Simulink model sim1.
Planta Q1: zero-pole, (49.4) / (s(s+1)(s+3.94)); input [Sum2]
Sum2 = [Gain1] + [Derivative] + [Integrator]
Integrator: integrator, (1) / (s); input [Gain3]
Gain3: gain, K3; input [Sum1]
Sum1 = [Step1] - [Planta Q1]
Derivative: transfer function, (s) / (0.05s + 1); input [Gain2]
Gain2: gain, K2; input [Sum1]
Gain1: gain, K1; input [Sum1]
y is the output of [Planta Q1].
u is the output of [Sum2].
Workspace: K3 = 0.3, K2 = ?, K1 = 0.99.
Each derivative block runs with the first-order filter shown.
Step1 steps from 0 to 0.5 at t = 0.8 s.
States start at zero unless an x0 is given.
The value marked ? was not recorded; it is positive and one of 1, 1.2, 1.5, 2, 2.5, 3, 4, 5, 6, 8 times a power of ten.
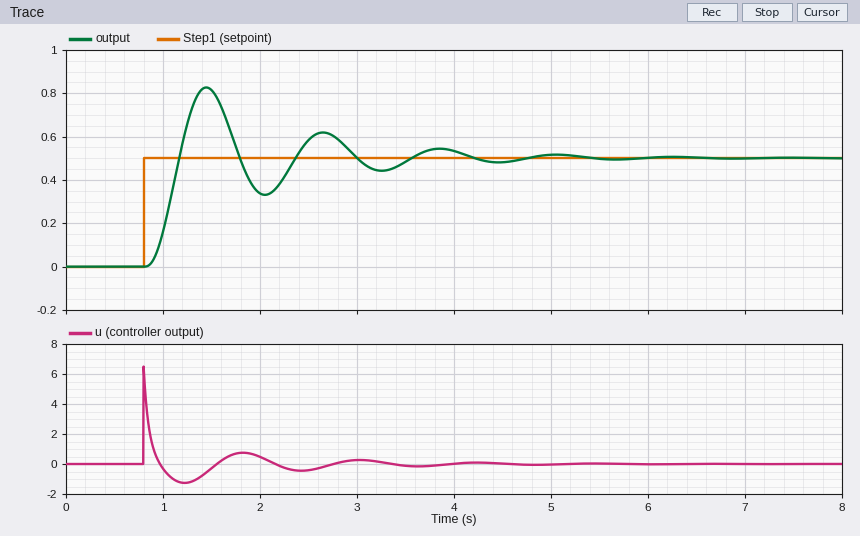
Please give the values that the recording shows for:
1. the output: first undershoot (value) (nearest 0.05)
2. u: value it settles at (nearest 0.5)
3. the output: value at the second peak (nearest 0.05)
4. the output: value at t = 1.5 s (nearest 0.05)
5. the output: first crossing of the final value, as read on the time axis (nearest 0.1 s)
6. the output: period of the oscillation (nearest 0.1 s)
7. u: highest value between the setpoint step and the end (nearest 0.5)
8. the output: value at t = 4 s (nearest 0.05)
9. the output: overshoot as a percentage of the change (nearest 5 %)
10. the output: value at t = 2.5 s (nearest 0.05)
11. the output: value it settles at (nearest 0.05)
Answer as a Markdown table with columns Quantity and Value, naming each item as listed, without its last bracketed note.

| Quantity | Value |
|---|---|
| the output: first undershoot (value) | 0.35 |
| u: value it settles at | 0.0 |
| the output: value at the second peak | 0.60 |
| the output: value at t = 1.5 s | 0.80 |
| the output: first crossing of the final value, as read on the time axis | 1.2 s |
| the output: period of the oscillation | 1.2 s |
| u: highest value between the setpoint step and the end | 6.5 |
| the output: value at t = 4 s | 0.55 |
| the output: overshoot as a percentage of the change | 65 % |
| the output: value at t = 2.5 s | 0.60 |
| the output: value it settles at | 0.50 |
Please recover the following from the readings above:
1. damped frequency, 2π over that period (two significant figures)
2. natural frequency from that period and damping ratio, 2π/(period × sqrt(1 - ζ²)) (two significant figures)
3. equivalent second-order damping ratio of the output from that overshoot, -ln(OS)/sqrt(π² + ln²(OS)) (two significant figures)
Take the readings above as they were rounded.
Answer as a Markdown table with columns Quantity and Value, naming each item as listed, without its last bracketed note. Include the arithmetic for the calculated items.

| Quantity | Value |
|---|---|
| damped frequency, 2π over that period | 2π / 1.2 = 5.2 rad/s |
| natural frequency from that period and damping ratio, 2π/(period × sqrt(1 - ζ²)) | 2π / (1.2 × sqrt(1 - 0.14²)) = 5.3 rad/s |
| equivalent second-order damping ratio of the output from that overshoot, -ln(OS)/sqrt(π² + ln²(OS)) | ln(0.65) = -0.431; 0.431 / sqrt(9.870 + 0.186) = 0.14 |
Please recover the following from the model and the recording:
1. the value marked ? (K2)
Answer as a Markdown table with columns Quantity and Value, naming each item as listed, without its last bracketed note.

| Quantity | Value |
|---|---|
| the value marked ? | 0.6 |
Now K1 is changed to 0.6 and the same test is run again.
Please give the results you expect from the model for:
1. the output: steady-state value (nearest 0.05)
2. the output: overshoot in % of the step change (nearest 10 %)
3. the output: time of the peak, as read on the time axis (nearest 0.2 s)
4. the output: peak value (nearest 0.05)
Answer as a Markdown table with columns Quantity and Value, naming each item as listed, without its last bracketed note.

| Quantity | Value |
|---|---|
| the output: steady-state value | 0.50 |
| the output: overshoot in % of the step change | 50 % |
| the output: time of the peak, as read on the time axis | 1.4 s |
| the output: peak value | 0.75 |
